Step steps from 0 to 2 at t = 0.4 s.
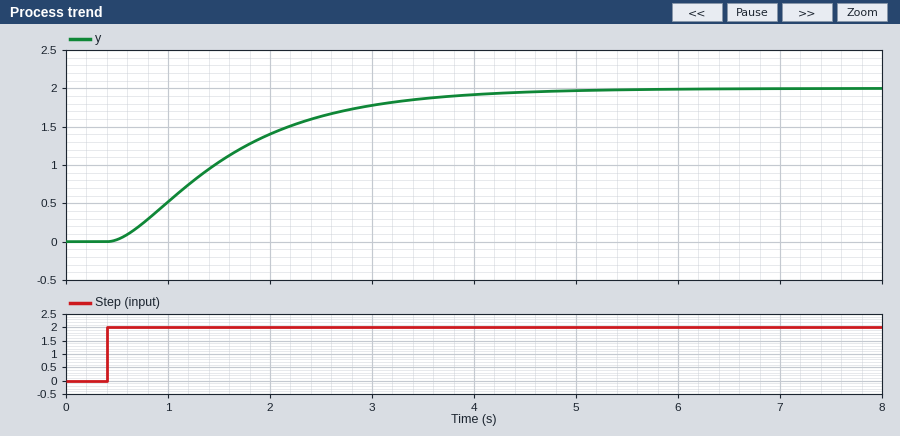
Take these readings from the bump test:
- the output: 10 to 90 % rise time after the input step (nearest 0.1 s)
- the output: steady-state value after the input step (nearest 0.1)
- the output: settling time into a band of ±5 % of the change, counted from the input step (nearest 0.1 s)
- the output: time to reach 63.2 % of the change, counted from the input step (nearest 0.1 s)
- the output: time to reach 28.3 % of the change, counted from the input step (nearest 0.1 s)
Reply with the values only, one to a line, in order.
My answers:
2.4 s
2.0
3.4 s
1.4 s
0.6 s
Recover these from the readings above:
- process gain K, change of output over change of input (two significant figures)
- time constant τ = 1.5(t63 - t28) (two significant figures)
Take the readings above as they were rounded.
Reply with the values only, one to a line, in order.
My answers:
1.0
1.2 s
